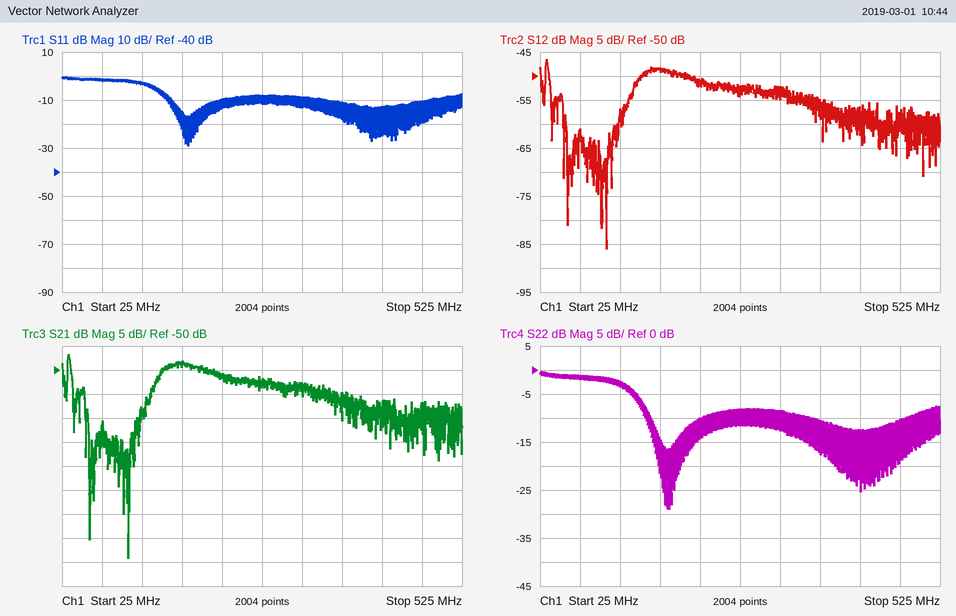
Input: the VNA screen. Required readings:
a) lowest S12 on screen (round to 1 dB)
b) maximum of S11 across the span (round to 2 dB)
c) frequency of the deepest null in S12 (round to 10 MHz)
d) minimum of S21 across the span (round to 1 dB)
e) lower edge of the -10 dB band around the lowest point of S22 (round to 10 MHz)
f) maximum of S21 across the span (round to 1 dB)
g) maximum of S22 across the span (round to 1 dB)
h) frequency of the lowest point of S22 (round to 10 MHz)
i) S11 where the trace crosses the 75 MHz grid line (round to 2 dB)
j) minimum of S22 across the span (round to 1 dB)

-86 dB
0 dB
110 MHz
-89 dB
160 MHz
-47 dB
0 dB
190 MHz
-2 dB
-29 dB
